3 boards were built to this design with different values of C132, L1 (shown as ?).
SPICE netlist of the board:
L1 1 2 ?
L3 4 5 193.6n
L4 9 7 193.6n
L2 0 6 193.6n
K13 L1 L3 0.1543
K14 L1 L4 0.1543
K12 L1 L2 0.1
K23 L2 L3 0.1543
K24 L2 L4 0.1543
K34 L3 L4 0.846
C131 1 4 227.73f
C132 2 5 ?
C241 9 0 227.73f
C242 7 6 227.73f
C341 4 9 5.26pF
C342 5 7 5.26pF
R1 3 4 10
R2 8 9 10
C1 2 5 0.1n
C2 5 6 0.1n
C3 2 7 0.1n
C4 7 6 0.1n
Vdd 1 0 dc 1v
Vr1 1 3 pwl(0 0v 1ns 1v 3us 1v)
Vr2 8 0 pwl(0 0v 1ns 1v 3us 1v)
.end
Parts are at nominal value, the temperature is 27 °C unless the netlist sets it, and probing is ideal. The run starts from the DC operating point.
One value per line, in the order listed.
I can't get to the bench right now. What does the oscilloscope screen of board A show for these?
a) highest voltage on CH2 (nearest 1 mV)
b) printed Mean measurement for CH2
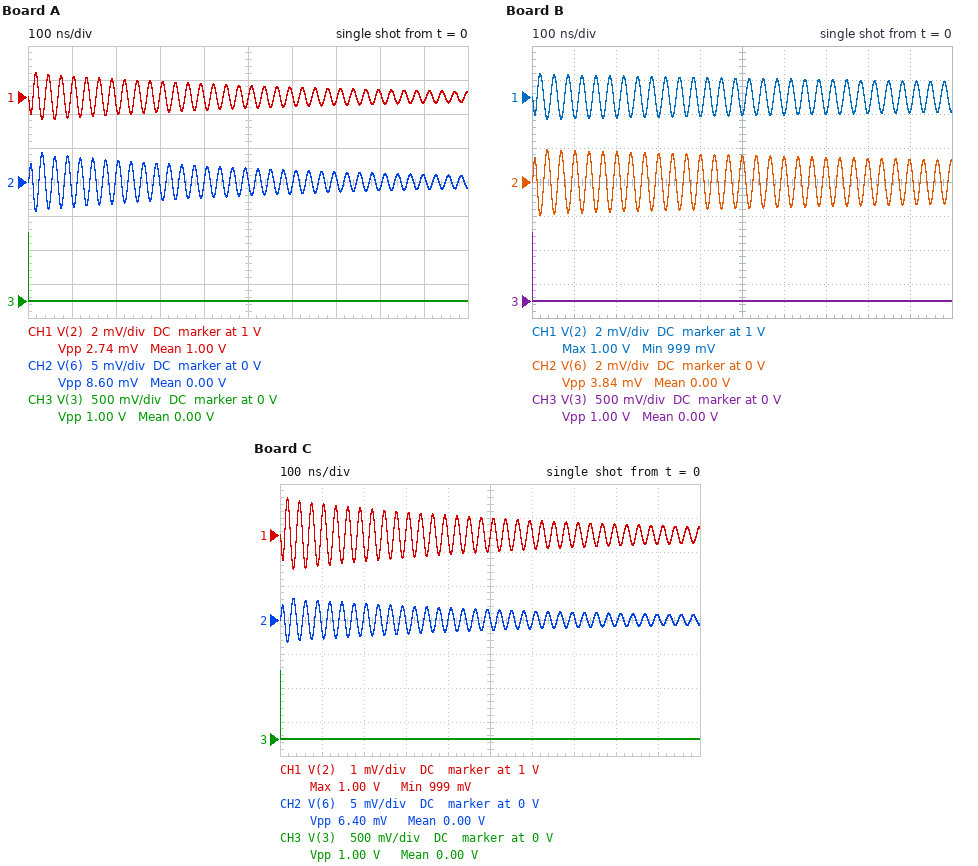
4 mV
0.00 V
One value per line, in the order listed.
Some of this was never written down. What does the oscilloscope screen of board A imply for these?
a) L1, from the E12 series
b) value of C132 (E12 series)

56 nH
680 fF
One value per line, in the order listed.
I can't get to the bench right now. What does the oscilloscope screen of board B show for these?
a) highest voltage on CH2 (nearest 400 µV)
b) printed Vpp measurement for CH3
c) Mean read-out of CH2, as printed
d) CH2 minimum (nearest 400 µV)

2.0 mV
1.00 V
0.00 V
-2.0 mV
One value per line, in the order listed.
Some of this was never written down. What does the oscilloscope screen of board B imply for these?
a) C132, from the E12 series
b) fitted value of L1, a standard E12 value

330 fF
120 nH
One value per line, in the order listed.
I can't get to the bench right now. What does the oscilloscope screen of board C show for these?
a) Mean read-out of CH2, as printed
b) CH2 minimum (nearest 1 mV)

0.00 V
-3 mV
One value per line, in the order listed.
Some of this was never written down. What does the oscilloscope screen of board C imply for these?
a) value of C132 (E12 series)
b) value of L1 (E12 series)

470 fF
56 nH
